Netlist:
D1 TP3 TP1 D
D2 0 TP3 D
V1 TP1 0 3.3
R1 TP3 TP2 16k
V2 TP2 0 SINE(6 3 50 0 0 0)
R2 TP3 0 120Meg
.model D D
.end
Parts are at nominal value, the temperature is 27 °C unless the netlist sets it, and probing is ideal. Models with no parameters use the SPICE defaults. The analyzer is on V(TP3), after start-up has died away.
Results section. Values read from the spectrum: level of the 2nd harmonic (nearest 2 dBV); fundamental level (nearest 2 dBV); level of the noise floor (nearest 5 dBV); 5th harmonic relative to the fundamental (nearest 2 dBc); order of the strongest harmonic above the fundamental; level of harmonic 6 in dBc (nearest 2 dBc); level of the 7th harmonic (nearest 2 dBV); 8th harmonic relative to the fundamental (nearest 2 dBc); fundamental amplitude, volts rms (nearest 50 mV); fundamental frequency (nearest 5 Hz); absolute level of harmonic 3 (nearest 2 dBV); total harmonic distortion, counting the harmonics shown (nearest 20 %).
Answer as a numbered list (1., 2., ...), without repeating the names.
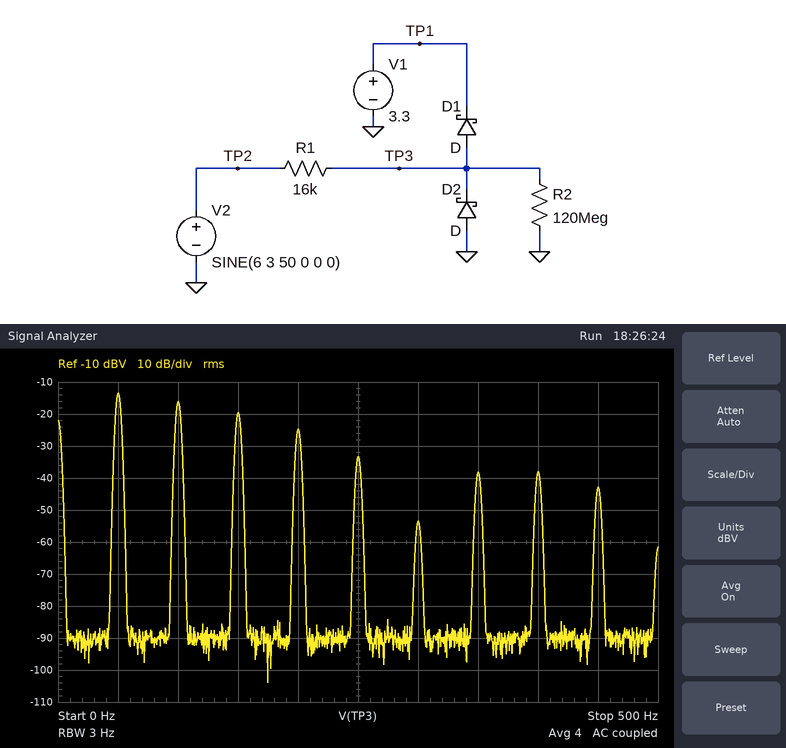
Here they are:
1. -16 dBV
2. -14 dBV
3. -90 dBV
4. -20 dBc
5. 2
6. -40 dBc
7. -38 dBV
8. -24 dBc
9. 200 mV
10. 50 Hz
11. -20 dBV
12. 100 %
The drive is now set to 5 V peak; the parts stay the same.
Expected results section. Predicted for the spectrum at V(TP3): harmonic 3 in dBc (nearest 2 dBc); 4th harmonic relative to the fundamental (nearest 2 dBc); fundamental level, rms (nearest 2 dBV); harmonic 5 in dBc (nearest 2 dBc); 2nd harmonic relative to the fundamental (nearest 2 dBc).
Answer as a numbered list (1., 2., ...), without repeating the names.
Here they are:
1. -12 dBc
2. -40 dBc
3. -2 dBV
4. -22 dBc
5. -4 dBc
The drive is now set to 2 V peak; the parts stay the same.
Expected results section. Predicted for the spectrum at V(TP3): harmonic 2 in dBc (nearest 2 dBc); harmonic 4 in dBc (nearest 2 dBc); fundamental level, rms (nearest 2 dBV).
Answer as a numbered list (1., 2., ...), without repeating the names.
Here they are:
1. -10 dBc
2. -24 dBc
3. -32 dBV
